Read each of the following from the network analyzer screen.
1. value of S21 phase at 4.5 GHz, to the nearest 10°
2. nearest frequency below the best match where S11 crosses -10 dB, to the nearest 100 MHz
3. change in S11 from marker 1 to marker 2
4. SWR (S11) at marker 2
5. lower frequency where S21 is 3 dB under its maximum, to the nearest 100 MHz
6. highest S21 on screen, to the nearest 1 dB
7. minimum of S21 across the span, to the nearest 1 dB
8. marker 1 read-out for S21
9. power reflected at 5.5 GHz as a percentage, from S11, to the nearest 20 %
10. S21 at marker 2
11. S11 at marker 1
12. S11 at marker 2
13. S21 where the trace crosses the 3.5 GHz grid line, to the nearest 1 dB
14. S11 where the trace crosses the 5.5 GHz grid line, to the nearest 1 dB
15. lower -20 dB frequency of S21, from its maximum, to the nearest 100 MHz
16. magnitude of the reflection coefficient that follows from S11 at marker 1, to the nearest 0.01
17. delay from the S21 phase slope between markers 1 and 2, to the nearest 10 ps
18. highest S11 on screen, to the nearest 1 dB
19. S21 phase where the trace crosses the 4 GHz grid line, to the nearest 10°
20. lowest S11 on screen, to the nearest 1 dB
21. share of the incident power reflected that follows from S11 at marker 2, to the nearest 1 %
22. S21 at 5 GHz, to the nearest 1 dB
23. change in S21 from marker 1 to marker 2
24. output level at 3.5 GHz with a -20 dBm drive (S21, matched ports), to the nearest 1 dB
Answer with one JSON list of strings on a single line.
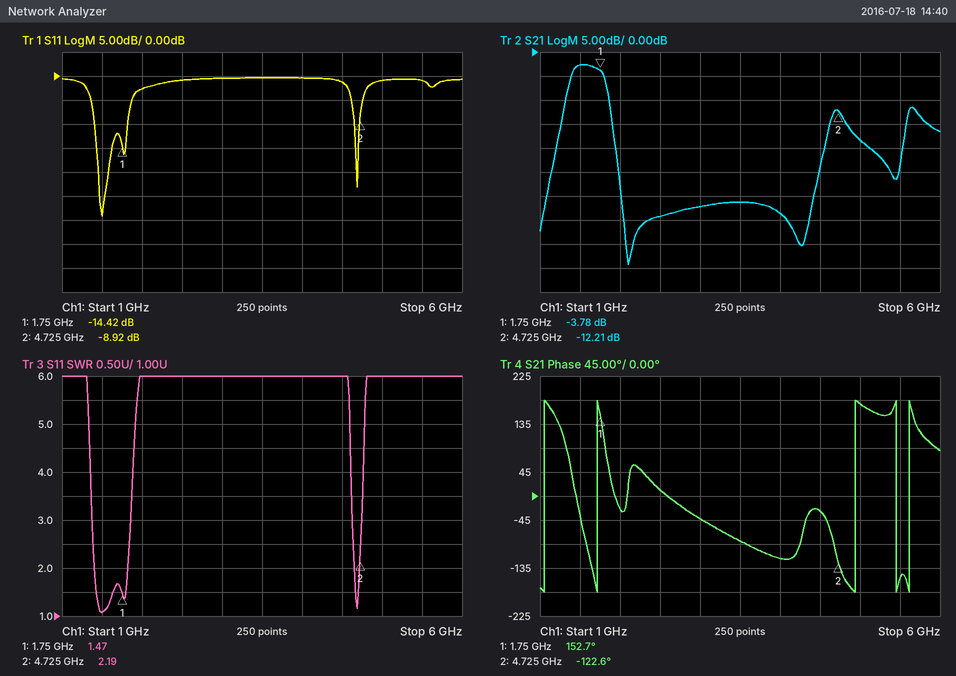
["-30°", "1.4 GHz", "5.50 dB", "2.19", "1.4 GHz", "-3 dB", "-44 dB", "-3.78 dB", "80 %", "-12.21 dB", "-14.42 dB", "-8.92 dB", "-31 dB", "-1 dB", "1.2 GHz", "0.19", "260 ps", "0 dB", "-120°", "-29 dB", "13 %", "-18 dB", "-8.43 dB", "-51 dBm"]
